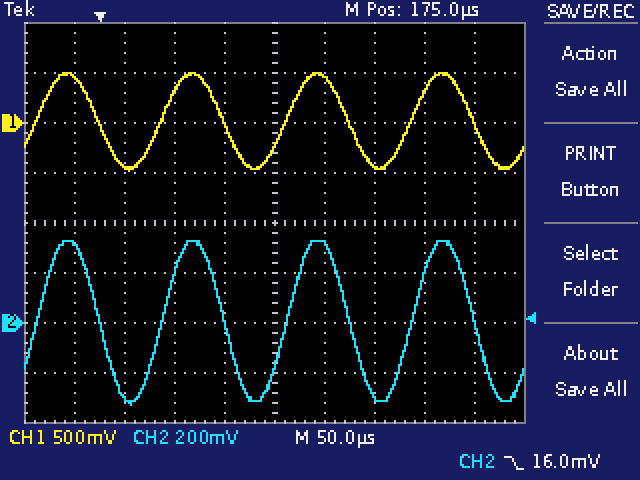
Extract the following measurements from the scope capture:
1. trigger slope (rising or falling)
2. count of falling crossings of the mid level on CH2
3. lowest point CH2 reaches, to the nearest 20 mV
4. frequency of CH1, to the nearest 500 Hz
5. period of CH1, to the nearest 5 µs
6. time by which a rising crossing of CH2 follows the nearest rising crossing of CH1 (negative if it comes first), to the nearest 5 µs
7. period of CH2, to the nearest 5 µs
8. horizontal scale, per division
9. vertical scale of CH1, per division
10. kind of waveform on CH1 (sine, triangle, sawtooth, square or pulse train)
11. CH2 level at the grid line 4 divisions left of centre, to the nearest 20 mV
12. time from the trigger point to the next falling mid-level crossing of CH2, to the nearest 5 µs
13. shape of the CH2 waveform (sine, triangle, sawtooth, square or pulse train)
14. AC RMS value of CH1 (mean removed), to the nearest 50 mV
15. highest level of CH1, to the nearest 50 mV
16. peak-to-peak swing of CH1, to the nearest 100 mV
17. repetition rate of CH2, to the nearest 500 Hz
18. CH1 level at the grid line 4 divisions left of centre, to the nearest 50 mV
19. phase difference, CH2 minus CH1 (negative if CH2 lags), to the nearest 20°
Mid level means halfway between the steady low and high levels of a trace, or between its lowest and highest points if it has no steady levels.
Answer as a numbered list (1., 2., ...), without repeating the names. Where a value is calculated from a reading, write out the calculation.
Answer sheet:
1. falling
2. 4
3. -320 mV
4. 1 / 125 µs ≈ 8.0 kHz
5. 125 µs
6. 0 µs
7. 125 µs
8. 50 µs
9. 500 mV
10. sine
11. 320 mV
12. 125 µs
13. sine
14. 1.00 V / (2√2) ≈ 354 mV, so 350 mV to the nearest 50 mV
15. 500 mV
16. 1.00 V
17. 1 / 125 µs ≈ 8.0 kHz
18. 450 mV
19. −360° × (0 µs) / 125 µs ≈ 0°
